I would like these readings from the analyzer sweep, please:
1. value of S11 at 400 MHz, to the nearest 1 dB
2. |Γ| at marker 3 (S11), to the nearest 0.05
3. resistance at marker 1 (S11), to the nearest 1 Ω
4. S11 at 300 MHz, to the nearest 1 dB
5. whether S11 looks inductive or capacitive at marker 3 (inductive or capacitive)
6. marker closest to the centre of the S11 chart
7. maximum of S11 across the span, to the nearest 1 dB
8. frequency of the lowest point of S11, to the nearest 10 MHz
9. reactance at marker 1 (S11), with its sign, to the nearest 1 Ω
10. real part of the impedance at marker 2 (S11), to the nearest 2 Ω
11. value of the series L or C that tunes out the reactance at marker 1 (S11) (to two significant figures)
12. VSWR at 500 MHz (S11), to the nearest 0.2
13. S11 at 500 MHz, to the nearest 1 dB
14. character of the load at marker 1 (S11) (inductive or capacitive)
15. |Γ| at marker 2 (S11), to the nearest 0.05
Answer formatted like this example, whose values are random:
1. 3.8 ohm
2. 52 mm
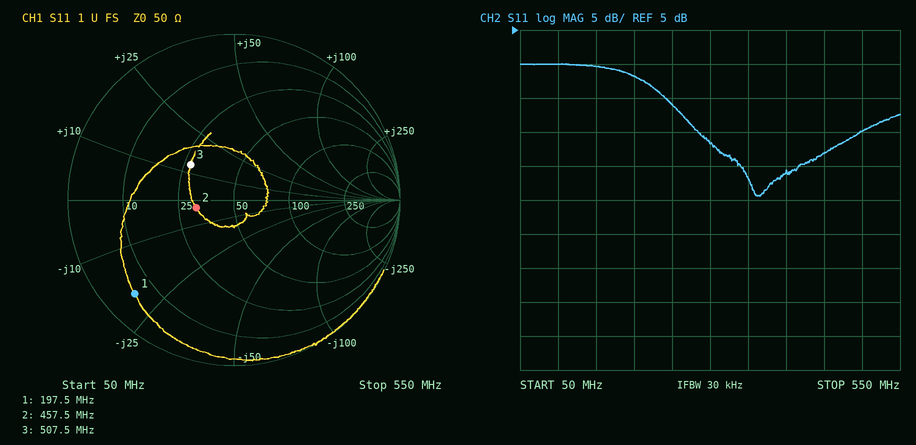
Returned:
1. -16 dB
2. 0.35
3. 6 Ω
4. -12 dB
5. inductive
6. marker 2
7. 0 dB
8. 360 MHz
9. -20 Ω
10. 32 Ω
11. 16 nH
12. 2.0
13. -10 dB
14. capacitive
15. 0.25
